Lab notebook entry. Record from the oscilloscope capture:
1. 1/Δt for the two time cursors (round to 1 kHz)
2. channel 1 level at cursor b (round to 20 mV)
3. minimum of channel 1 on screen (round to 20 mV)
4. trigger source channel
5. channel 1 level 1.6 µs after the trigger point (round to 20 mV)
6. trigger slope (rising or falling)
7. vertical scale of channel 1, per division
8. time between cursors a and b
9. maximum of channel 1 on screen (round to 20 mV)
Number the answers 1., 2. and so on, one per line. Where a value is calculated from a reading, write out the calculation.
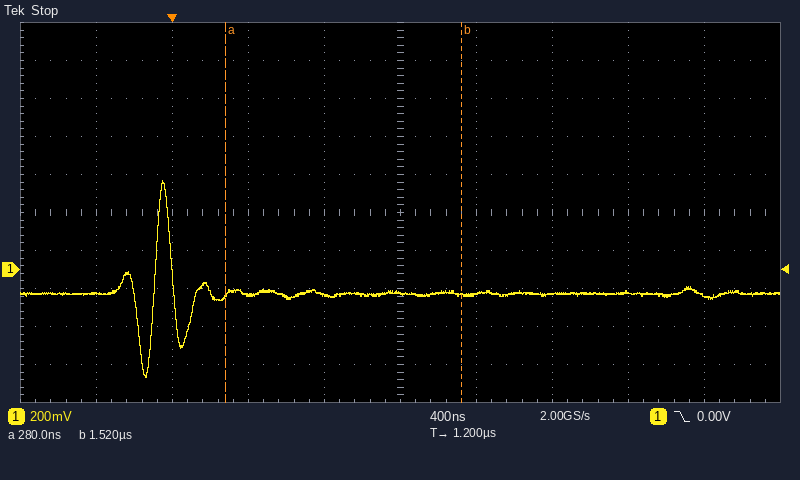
1. 1 / 1.24 µs ≈ 806 kHz
2. -140 mV
3. -560 mV
4. channel 1
5. -120 mV
6. falling
7. 200 mV
8. 1.52 µs − (280 ns) = 1.24 µs
9. 460 mV
